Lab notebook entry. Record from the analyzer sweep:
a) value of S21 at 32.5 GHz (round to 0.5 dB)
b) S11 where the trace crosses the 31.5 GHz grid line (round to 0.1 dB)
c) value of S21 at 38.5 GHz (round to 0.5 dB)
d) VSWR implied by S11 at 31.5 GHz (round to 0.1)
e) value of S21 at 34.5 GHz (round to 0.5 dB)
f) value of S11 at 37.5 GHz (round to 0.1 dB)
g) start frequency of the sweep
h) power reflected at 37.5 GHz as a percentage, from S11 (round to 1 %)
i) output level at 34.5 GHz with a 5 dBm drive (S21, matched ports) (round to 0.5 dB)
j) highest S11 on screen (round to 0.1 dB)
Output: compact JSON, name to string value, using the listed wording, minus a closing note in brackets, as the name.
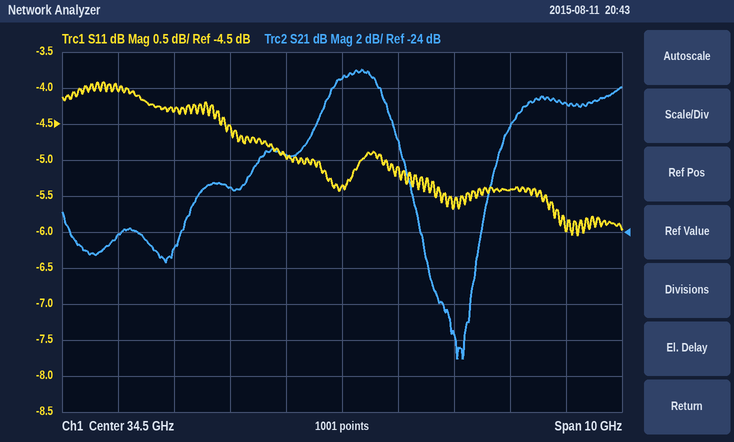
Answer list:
{"value of S21 at 32.5 GHz": "-21.5 dB", "S11 where the trace crosses the 31.5 GHz grid line": "-4.3 dB", "value of S21 at 38.5 GHz": "-17.0 dB", "VSWR implied by S11 at 31.5 GHz": "4.1", "value of S21 at 34.5 GHz": "-15.5 dB", "value of S11 at 37.5 GHz": "-5.4 dB", "start frequency of the sweep": "29.5 GHz", "power reflected at 37.5 GHz as a percentage, from S11": "29 %", "output level at 34.5 GHz with a 5 dBm drive (S21, matched ports)": "-10.5 dBm", "highest S11 on screen": "-3.9 dB"}
